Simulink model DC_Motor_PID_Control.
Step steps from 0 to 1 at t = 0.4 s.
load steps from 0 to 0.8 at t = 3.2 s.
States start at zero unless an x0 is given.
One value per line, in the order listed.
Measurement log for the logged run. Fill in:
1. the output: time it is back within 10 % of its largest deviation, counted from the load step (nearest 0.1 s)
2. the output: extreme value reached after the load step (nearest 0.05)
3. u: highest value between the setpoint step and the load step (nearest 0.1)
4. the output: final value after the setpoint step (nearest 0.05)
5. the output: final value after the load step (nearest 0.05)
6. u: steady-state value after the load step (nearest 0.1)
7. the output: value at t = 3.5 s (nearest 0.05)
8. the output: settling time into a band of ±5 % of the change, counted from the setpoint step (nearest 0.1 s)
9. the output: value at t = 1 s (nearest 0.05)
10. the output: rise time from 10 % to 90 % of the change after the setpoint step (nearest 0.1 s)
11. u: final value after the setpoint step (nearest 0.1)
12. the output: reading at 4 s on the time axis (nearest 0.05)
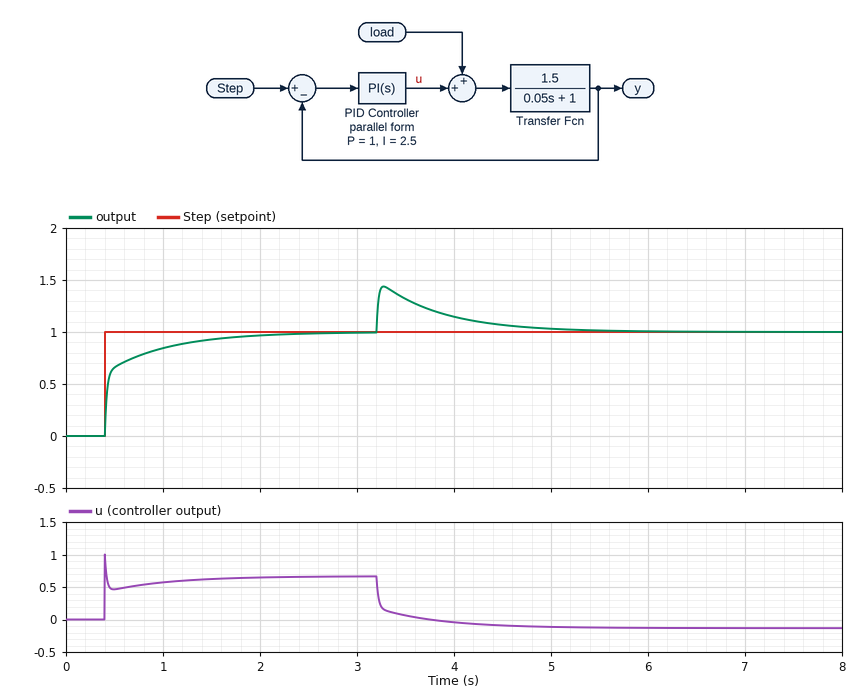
1.6 s
1.45
1.0
1.00
1.00
-0.1
1.30
1.3 s
0.85
0.9 s
0.7
1.15
